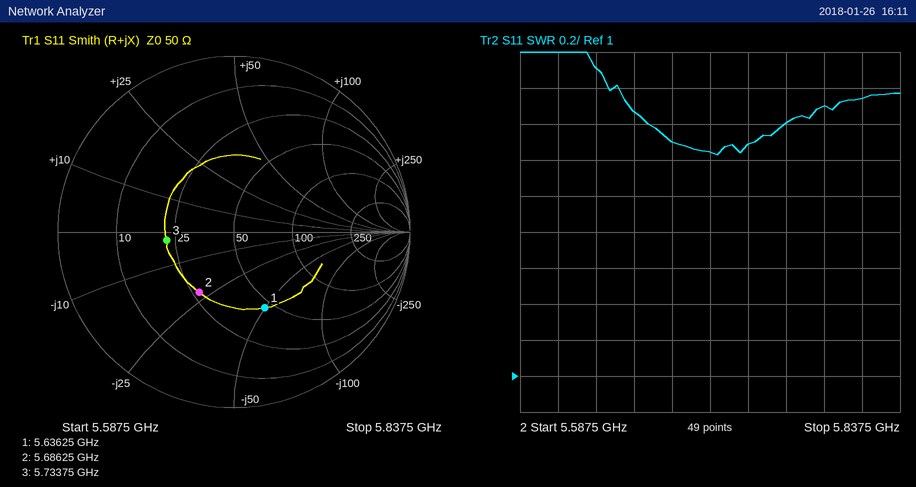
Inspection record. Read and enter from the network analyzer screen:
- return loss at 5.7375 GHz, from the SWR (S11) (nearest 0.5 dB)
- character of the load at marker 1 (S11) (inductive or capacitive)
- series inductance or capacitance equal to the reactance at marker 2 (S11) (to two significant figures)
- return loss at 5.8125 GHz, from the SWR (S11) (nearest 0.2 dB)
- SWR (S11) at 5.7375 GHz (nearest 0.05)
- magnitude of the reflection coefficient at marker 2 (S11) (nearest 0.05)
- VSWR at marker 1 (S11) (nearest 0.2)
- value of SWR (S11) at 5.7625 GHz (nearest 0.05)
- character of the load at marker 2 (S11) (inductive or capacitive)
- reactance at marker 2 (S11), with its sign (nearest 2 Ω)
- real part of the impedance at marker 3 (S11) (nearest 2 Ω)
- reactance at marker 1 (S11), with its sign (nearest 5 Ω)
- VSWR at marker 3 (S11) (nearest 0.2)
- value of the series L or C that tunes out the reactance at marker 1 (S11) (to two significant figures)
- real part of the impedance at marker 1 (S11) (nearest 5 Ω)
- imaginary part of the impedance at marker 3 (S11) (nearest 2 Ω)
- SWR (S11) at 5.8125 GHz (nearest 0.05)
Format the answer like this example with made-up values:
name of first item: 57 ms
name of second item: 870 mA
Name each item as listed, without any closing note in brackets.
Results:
return loss at 5.7375 GHz, from the SWR (S11): 8.0 dB
character of the load at marker 1 (S11): capacitive
series inductance or capacitance equal to the reactance at marker 2 (S11): 1.3 pF
return loss at 5.8125 GHz, from the SWR (S11): 7.2 dB
SWR (S11) at 5.7375 GHz: 2.30
magnitude of the reflection coefficient at marker 2 (S11): 0.40
VSWR at marker 1 (S11): 2.8
value of SWR (S11) at 5.7625 GHz: 2.40
character of the load at marker 2 (S11): capacitive
reactance at marker 2 (S11), with its sign: -22 Ω
real part of the impedance at marker 3 (S11): 22 Ω
reactance at marker 1 (S11), with its sign: -50 Ω
VSWR at marker 3 (S11): 2.2
value of the series L or C that tunes out the reactance at marker 1 (S11): 1.4 nH
real part of the impedance at marker 1 (S11): 45 Ω
imaginary part of the impedance at marker 3 (S11): -2 Ω
SWR (S11) at 5.8125 GHz: 2.55
